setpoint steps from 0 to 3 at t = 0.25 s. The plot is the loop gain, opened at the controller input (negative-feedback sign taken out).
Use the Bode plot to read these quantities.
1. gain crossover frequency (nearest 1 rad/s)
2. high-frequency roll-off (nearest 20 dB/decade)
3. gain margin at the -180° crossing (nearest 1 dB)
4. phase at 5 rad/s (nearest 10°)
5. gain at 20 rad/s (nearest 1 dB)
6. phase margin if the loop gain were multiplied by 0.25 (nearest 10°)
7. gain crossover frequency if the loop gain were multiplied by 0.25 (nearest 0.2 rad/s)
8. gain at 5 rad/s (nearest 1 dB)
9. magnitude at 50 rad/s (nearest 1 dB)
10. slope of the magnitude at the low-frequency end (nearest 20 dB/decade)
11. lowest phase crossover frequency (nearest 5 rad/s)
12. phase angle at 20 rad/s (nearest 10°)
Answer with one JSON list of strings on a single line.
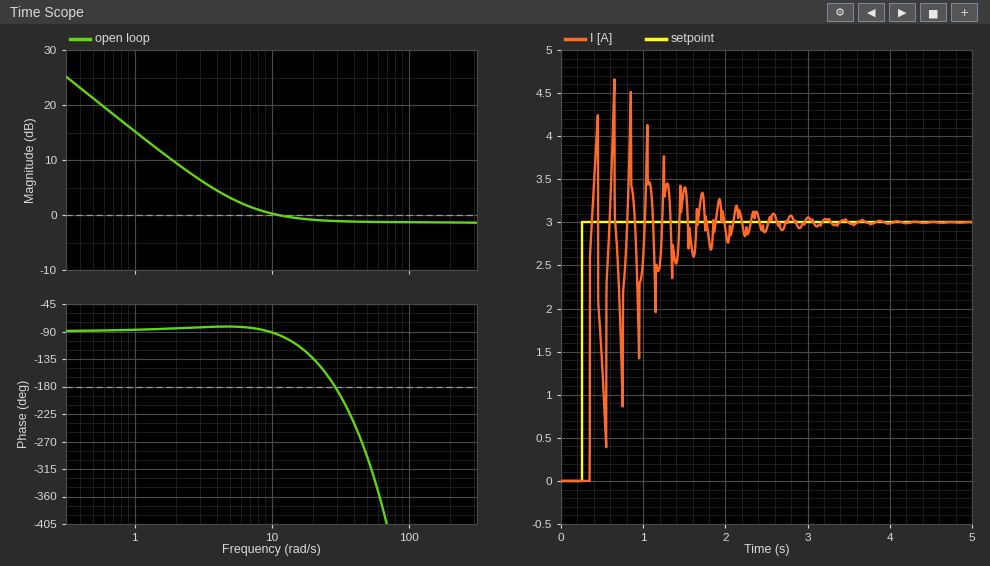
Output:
["11 rad/s", "0 dB/decade", "1 dB", "-80°", "-1 dB", "90°", "1.4 rad/s", "3 dB", "-1 dB", "-20 dB/decade", "30 rad/s", "-130°"]
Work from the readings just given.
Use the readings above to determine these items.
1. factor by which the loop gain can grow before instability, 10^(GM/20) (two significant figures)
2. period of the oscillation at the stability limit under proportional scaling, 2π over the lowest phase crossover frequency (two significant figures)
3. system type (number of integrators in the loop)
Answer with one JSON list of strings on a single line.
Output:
["1.1", "0.21 s", "1"]
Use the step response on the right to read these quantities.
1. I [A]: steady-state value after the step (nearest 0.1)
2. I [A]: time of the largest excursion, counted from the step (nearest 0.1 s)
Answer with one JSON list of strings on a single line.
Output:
["3.0", "0.4 s"]
